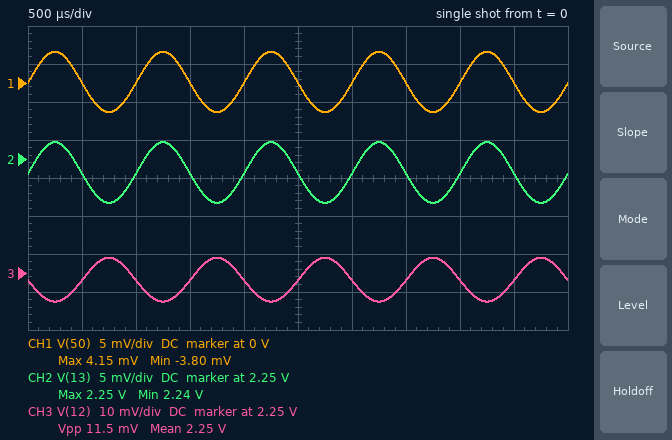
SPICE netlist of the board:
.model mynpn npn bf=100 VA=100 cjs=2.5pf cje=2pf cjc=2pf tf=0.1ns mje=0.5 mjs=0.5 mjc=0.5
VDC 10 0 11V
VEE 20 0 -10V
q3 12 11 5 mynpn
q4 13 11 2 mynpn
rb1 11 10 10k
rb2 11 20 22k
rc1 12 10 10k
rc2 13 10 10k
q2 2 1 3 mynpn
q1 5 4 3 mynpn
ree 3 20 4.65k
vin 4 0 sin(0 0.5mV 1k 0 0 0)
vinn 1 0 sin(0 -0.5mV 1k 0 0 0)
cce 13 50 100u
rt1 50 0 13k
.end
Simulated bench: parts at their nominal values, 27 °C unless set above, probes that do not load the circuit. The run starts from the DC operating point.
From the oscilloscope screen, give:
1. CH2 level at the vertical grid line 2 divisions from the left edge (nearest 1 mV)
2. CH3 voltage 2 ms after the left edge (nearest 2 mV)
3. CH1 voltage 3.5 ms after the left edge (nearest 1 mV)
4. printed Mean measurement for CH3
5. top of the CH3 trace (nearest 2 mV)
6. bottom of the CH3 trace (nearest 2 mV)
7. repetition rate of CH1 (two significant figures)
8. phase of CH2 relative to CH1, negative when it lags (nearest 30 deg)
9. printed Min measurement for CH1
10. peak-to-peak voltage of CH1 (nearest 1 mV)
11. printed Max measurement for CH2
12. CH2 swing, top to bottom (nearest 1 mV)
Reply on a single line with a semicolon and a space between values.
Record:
2.248 V; 2.248 V; 0 V; 2.25 V; 2.254 V; 2.242 V; 1.0 kHz; 0 deg; -3.80 mV; 8 mV; 2.25 V; 8 mV
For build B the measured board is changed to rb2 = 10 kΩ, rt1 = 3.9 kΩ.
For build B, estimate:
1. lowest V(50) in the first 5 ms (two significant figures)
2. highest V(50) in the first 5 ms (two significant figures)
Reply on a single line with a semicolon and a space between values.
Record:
-53 mV; 53 mV
